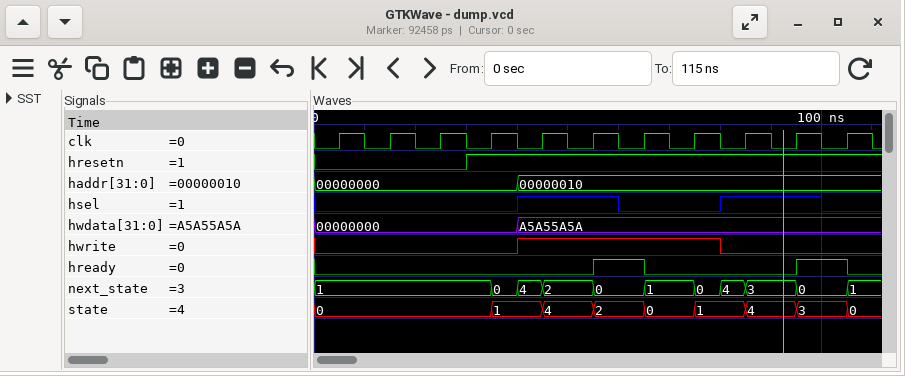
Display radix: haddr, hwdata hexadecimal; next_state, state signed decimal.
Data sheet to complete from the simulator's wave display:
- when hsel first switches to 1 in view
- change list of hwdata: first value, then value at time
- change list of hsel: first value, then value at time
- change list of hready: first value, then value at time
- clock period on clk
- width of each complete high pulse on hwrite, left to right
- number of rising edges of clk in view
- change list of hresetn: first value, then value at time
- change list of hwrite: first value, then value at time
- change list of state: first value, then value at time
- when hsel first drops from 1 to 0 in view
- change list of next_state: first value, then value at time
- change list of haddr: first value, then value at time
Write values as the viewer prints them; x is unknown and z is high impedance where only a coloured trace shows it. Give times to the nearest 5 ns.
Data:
40 ns
00000000, A5A55A5A at 40 ns
0, 1 at 40 ns, 0 at 60 ns, 1 at 80 ns, 0 at 100 ns
0, 1 at 55 ns, 0 at 65 ns, 1 at 95 ns, 0 at 105 ns
10 ns
40 ns
11
0, 1 at 30 ns
0, 1 at 40 ns, 0 at 80 ns
0, 1 at 35 ns, 4 at 45 ns, 2 at 55 ns, 0 at 65 ns, 1 at 75 ns, 4 at 85 ns, 3 at 95 ns, 0 at 105 ns
60 ns
1, 0 at 35 ns, 4 at 40 ns, 2 at 45 ns, 0 at 55 ns, 1 at 65 ns, 0 at 75 ns, 4 at 80 ns, 3 at 85 ns, 0 at 95 ns, 1 at 105 ns
00000000, 00000010 at 40 ns
